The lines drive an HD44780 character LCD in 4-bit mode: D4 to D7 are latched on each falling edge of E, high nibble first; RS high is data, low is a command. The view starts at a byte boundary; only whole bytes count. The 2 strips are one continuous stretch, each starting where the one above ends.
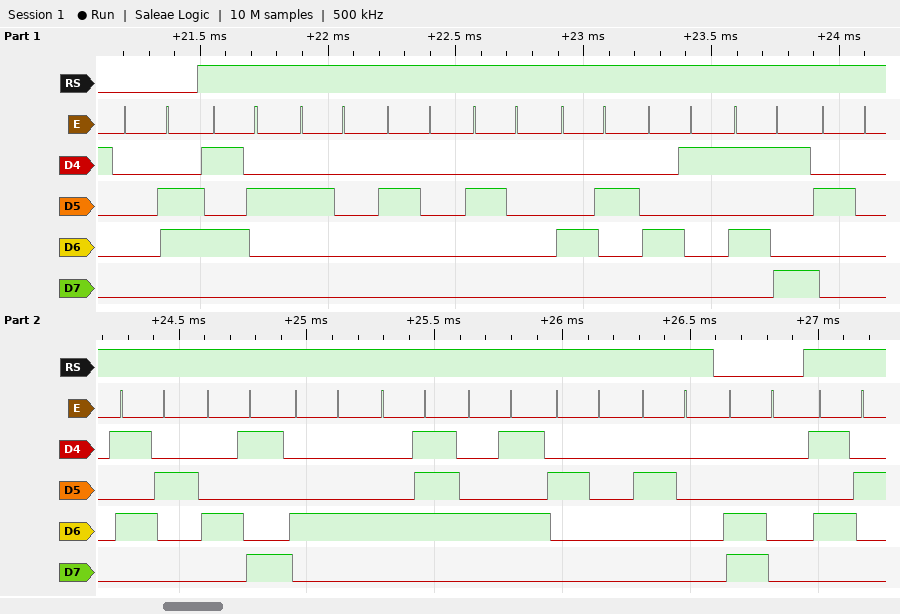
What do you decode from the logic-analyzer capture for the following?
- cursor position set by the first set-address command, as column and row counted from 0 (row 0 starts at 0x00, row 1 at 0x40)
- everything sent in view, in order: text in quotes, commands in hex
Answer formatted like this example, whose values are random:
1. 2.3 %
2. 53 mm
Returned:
1. column 0, row 1
2. 0x06 "R   BAY RIDGE  " 0xC0 "R"
